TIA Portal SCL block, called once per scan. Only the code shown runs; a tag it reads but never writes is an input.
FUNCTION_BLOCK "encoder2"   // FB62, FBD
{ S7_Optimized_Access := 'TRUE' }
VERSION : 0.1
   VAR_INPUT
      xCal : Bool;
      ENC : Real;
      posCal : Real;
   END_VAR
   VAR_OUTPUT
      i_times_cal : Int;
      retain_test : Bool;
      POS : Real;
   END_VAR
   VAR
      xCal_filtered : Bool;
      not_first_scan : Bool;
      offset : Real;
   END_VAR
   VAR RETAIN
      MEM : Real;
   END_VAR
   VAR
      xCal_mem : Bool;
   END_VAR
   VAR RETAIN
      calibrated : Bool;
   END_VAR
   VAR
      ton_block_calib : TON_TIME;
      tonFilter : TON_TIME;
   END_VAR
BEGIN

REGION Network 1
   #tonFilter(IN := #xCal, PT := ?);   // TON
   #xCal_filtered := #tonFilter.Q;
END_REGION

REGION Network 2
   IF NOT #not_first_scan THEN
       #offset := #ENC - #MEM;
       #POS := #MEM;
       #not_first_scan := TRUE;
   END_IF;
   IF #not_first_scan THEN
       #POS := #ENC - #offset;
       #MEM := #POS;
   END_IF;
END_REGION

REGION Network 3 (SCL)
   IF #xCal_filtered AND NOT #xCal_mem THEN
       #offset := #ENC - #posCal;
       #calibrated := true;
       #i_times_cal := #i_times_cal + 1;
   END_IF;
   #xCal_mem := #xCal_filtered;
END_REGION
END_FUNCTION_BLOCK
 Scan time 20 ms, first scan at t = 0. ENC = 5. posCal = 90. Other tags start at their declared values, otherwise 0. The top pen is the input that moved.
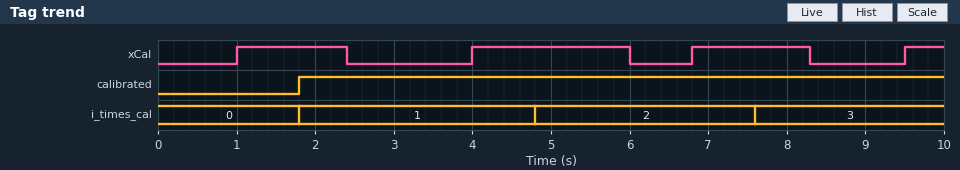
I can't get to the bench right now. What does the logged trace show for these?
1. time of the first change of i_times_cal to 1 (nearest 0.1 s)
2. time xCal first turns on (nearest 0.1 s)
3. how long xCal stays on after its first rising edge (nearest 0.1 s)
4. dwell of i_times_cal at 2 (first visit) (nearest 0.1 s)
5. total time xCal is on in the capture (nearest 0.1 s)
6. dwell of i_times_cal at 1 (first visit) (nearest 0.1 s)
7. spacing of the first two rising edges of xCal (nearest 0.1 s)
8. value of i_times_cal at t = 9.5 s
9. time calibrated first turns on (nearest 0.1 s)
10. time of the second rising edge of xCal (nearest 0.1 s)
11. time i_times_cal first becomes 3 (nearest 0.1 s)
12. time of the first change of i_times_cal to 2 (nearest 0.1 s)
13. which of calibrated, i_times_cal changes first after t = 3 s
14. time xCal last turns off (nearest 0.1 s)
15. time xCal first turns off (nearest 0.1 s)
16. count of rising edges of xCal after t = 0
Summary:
1.8 s
1.0 s
1.4 s
2.8 s
5.4 s
3.0 s
3.0 s
3
1.8 s
4.0 s
7.6 s
4.8 s
i_times_cal
8.3 s
2.4 s
4
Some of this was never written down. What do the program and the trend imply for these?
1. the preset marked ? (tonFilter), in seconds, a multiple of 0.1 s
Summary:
0.8 s
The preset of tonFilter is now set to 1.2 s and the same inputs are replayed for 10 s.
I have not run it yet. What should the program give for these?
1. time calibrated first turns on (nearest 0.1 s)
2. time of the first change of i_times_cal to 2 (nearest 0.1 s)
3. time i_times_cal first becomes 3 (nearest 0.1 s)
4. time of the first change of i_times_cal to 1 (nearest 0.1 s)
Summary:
2.2 s
5.2 s
8.0 s
2.2 s
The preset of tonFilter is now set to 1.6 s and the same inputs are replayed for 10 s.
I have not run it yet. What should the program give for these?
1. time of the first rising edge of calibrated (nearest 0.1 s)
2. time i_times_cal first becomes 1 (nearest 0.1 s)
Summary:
5.6 s
5.6 s
